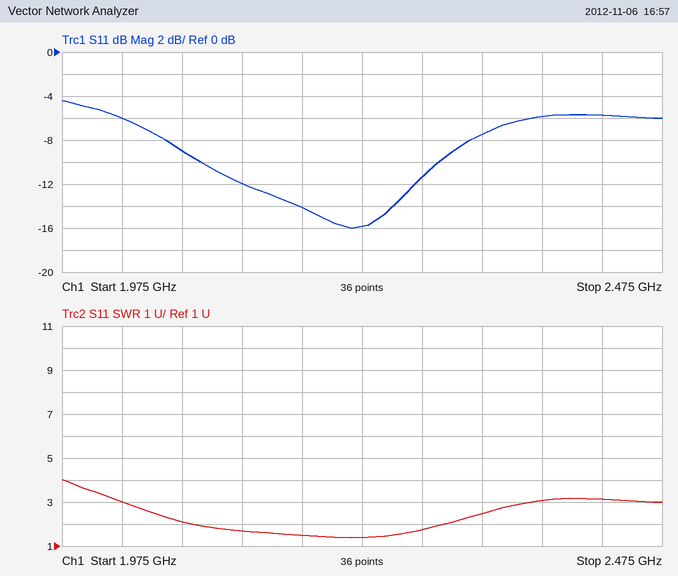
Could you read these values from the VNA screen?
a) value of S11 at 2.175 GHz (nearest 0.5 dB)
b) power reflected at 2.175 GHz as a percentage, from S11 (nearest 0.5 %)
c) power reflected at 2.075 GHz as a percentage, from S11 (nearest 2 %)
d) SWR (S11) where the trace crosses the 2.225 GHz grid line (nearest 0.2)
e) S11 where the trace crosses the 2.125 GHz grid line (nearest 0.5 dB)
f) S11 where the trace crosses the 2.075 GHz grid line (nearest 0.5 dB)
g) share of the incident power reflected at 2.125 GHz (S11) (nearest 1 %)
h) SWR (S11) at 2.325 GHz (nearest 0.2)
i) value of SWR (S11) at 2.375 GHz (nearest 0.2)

-14.0 dB
4.0 %
12 %
1.4
-12.0 dB
-9.0 dB
6 %
2.4
3.0
